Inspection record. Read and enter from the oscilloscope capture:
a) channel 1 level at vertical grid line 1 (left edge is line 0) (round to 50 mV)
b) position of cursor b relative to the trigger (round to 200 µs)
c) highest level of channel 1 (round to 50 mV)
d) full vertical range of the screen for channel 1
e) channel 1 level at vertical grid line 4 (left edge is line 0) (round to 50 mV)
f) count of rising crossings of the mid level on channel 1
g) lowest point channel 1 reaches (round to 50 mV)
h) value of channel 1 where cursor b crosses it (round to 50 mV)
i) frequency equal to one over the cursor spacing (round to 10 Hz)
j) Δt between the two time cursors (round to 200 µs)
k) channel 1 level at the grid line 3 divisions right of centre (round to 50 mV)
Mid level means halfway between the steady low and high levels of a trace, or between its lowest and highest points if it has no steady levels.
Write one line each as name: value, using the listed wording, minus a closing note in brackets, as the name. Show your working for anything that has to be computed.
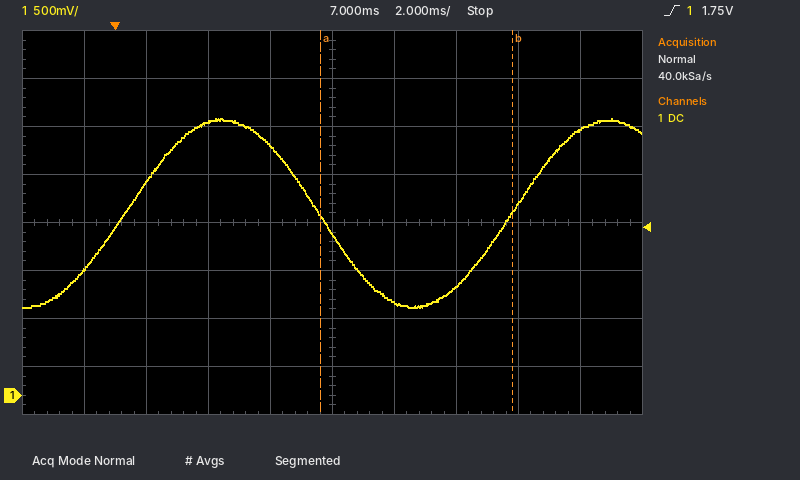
channel 1 level at vertical grid line 1 (left edge is line 0): 1.30 V
position of cursor b relative to the trigger: +12.8 ms
highest level of channel 1: 2.90 V
full vertical range of the screen for channel 1: 4 V
channel 1 level at vertical grid line 4 (left edge is line 0): 2.60 V
count of rising crossings of the mid level on channel 1: 2
lowest point channel 1 reaches: 900 mV
value of channel 1 where cursor b crosses it: 1.90 V
frequency equal to one over the cursor spacing: 1 / 6.2 ms ≈ 160 Hz
Δt between the two time cursors: 6.2 ms
channel 1 level at the grid line 3 divisions right of centre: 2.00 V
